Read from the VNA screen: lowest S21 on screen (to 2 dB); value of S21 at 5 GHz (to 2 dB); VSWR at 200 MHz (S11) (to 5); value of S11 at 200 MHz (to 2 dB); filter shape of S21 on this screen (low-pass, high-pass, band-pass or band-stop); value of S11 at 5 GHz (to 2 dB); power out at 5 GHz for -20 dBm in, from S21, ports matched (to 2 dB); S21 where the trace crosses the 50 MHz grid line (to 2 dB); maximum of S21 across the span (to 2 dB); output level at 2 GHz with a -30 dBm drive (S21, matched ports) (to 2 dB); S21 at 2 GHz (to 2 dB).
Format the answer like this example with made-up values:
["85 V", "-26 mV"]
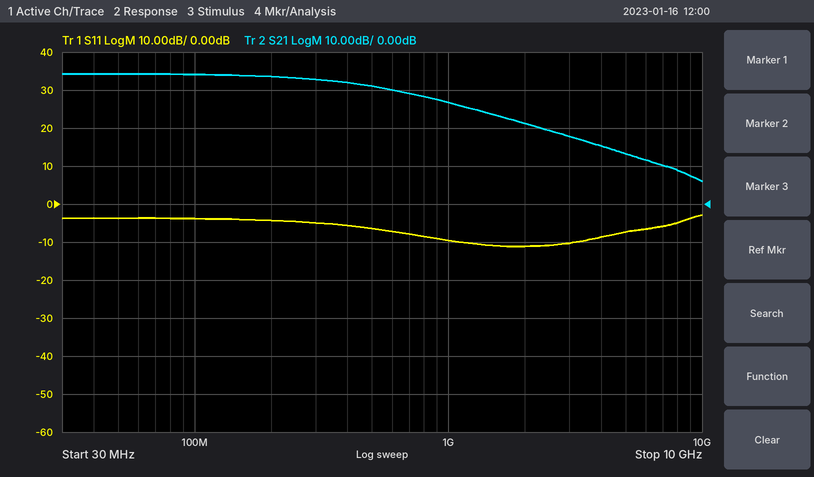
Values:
["6 dB", "14 dB", "5", "-4 dB", "low-pass", "-8 dB", "-6 dBm", "34 dB", "34 dB", "-8 dBm", "22 dB"]
